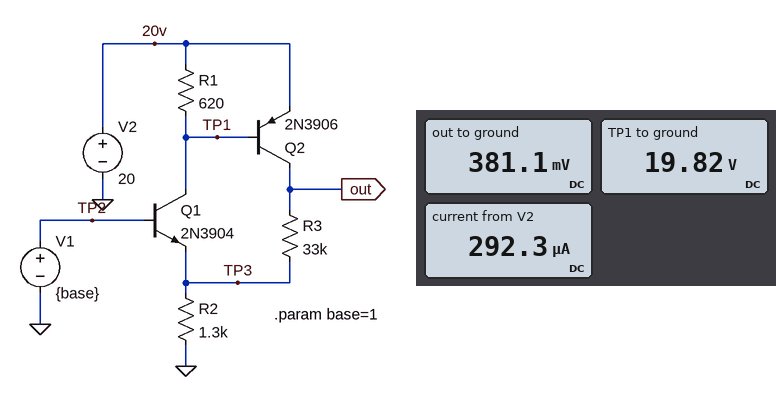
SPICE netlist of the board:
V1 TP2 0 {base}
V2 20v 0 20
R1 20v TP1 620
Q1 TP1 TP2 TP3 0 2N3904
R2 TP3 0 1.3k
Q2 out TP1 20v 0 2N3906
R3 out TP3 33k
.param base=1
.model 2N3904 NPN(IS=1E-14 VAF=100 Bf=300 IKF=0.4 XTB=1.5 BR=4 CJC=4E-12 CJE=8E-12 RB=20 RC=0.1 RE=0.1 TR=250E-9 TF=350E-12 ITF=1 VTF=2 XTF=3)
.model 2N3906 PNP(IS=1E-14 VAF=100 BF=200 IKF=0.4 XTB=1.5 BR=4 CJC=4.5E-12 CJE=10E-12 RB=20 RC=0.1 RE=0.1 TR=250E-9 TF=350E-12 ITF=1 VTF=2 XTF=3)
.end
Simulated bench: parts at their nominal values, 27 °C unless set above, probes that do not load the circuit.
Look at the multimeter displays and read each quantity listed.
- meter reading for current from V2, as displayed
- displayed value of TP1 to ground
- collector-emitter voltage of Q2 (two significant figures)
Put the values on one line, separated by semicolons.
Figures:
292.3 µA; 19.82 V; -20 V
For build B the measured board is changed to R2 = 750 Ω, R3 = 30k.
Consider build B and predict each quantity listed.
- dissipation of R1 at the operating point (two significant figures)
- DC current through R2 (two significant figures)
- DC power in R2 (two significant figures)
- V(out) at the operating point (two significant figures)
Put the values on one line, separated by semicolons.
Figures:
150 µW; 490 µA; 180 µW; 370 mV
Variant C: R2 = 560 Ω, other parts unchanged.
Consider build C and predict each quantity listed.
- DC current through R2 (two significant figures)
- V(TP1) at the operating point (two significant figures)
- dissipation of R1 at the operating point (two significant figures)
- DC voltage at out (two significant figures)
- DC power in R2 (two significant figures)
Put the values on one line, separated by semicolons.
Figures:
640 µA; 20 V; 260 µW; 360 mV; 230 µW
